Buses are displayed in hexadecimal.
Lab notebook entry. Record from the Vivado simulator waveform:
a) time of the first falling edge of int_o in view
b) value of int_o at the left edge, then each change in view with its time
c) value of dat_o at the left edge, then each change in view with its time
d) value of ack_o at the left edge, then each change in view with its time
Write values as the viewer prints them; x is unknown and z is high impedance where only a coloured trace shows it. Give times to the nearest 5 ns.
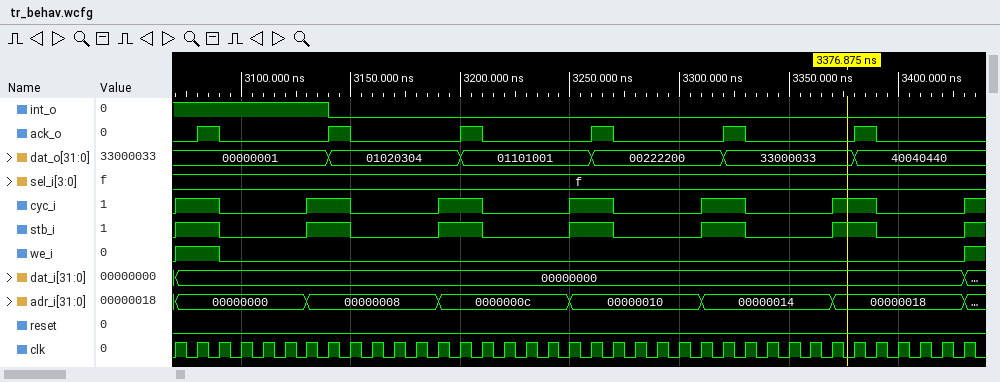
3140 ns
1, 0 at 3140 ns
00000001, 01020304 at 3140 ns, 01101001 at 3200 ns, 00222200 at 3260 ns, 33000033 at 3320 ns, 40040440 at 3380 ns
0, 1 at 3080 ns, 0 at 3090 ns, 1 at 3140 ns, 0 at 3150 ns, 1 at 3200 ns, 0 at 3210 ns, 1 at 3260 ns, 0 at 3270 ns, 1 at 3320 ns, 0 at 3330 ns, 1 at 3380 ns, 0 at 3390 ns
